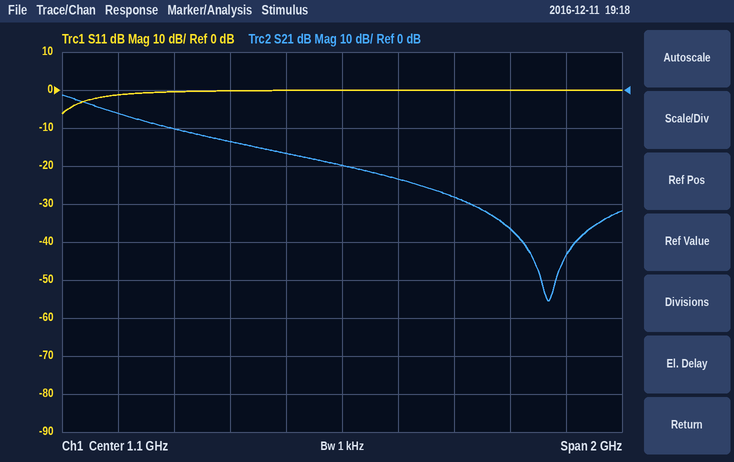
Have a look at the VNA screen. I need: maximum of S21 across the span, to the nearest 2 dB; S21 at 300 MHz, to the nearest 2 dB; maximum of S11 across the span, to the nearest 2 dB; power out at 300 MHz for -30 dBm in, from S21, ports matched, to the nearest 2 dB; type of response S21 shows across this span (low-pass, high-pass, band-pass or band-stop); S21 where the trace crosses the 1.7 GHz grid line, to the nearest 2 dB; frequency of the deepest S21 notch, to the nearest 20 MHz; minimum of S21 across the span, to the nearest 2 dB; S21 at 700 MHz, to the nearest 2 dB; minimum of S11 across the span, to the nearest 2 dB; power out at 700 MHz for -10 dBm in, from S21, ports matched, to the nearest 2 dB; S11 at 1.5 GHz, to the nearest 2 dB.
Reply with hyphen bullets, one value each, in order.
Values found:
- -2 dB
- -6 dB
- 0 dB
- -36 dBm
- low-pass
- -36 dB
- 1.84 GHz
- -56 dB
- -14 dB
- -6 dB
- -24 dBm
- 0 dB
